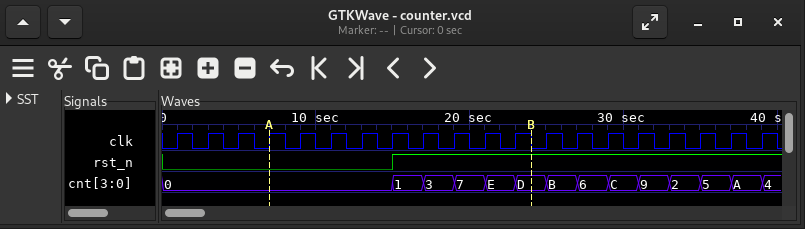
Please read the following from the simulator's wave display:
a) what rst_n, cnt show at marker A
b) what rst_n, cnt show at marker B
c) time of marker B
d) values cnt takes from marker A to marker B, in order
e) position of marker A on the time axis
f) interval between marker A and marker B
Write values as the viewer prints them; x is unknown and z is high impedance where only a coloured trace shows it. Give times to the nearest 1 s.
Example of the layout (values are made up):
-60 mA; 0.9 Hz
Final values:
rst_n=0, cnt=0; rst_n=1, cnt=D; 24 s; 0, 1, 3, 7, E, D; 7 s; 17 s
